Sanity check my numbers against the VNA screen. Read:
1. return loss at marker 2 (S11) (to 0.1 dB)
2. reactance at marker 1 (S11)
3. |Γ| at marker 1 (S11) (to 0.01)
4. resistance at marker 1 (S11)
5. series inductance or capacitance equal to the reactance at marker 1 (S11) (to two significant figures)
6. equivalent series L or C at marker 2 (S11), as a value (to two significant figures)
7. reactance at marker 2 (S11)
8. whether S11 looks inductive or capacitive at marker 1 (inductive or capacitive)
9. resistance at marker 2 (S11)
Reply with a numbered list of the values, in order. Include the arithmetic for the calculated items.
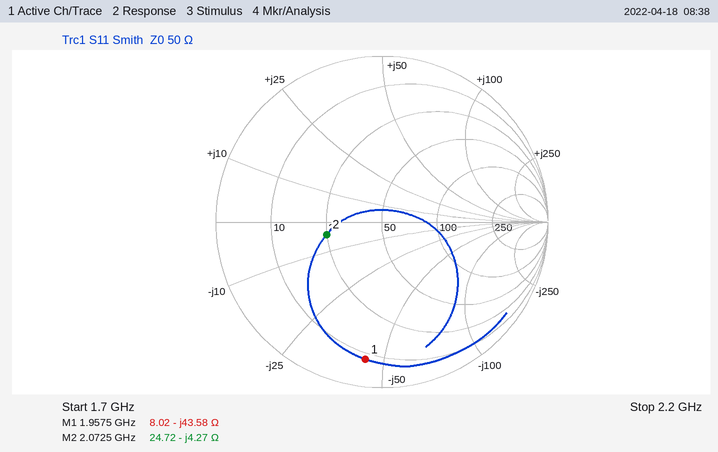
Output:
1. 9.3 dB
2. -43.58 Ω
3. 0.83
4. 8.02 Ω
5. C = 1/(2π × 1.9575 GHz × 43.58 Ω) ≈ 1.9 pF
6. C = 1/(2π × 2.0725 GHz × 4.27 Ω) ≈ 18 pF
7. -4.27 Ω
8. capacitive
9. 24.72 Ω
